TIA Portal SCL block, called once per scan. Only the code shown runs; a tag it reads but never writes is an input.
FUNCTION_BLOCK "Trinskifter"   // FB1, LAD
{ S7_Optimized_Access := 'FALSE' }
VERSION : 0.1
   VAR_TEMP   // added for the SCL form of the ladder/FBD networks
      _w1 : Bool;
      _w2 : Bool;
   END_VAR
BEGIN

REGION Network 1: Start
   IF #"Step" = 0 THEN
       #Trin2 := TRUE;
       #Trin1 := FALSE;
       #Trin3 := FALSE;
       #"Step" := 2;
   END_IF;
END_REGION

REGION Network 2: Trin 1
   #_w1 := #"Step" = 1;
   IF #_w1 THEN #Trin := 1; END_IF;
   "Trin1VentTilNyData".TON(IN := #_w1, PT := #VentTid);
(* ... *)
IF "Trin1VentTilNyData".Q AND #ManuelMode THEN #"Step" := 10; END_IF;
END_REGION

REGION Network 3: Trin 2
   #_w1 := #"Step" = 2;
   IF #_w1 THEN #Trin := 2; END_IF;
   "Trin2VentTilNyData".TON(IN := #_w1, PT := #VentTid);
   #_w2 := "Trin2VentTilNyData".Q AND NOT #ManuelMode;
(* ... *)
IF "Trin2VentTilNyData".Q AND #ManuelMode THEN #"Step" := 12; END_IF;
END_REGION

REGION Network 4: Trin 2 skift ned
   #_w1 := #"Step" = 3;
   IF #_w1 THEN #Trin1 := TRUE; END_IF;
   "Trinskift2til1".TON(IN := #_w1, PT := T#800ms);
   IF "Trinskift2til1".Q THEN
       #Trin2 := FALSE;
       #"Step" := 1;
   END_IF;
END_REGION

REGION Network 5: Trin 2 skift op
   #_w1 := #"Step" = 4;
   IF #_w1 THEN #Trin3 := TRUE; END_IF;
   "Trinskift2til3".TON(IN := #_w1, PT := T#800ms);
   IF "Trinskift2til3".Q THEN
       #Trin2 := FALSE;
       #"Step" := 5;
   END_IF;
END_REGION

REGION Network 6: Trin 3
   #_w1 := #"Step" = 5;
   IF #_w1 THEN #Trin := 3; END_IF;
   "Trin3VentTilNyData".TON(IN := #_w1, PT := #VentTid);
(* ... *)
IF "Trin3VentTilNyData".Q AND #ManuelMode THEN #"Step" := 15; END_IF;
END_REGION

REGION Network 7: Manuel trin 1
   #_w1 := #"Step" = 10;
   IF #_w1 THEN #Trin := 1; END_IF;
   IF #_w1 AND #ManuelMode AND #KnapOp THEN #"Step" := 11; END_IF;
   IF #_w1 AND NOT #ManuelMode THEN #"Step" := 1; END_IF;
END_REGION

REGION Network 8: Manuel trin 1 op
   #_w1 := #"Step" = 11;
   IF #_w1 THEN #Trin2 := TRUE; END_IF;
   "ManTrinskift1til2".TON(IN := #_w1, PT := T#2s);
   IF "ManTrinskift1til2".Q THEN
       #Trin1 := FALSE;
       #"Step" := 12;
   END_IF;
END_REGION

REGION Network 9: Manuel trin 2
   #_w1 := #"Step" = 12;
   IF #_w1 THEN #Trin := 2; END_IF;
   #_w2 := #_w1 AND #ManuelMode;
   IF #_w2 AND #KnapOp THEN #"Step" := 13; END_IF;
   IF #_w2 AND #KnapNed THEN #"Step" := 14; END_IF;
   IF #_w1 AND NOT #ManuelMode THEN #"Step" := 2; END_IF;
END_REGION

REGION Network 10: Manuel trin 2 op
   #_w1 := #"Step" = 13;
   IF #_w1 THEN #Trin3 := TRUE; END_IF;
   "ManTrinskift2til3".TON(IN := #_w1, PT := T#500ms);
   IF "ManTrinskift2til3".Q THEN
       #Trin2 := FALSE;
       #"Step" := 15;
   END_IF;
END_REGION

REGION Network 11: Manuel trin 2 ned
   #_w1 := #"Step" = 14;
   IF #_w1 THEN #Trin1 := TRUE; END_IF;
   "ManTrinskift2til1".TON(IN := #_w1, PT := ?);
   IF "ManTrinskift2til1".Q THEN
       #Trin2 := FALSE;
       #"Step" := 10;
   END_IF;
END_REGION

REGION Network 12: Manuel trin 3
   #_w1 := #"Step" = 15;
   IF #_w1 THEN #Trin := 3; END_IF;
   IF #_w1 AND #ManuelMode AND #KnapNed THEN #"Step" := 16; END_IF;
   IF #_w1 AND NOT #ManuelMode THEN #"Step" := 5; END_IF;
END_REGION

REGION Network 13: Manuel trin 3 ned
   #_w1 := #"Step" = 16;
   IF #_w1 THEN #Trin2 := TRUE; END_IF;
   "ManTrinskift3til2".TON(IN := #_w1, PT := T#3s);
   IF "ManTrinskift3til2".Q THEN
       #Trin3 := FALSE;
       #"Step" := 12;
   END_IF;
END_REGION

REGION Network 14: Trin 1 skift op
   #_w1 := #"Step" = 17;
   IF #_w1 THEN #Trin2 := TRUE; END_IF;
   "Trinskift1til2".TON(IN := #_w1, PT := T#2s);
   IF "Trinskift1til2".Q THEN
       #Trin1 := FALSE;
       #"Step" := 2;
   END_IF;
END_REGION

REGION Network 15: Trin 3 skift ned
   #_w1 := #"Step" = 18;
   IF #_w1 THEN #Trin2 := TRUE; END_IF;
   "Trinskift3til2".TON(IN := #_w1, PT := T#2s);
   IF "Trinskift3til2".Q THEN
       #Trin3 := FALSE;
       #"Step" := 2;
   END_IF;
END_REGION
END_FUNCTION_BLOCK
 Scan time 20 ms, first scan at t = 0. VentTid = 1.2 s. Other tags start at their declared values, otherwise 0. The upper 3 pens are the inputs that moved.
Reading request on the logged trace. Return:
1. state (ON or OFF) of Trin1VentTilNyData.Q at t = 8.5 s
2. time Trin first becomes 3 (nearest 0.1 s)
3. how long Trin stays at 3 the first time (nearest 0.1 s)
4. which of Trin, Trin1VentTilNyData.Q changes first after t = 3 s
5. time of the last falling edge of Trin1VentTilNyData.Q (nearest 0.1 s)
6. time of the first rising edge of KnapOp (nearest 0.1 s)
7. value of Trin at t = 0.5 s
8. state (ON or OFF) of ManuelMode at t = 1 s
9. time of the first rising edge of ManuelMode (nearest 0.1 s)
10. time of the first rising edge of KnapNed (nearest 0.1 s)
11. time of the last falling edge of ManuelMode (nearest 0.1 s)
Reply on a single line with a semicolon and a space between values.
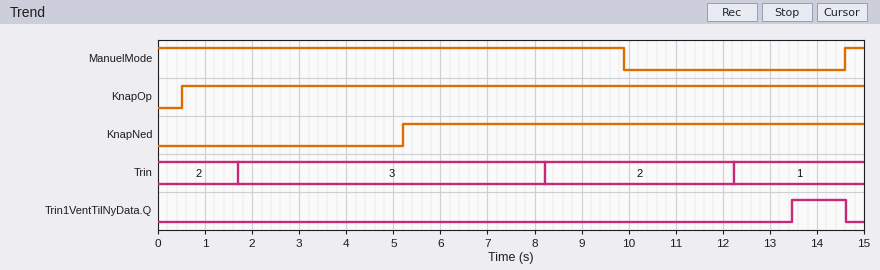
OFF; 1.7 s; 6.5 s; Trin; 14.6 s; 0.5 s; 2; ON; 14.6 s; 5.2 s; 9.9 s
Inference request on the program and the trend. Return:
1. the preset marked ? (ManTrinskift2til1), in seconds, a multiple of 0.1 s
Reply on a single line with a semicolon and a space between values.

4.0 s
